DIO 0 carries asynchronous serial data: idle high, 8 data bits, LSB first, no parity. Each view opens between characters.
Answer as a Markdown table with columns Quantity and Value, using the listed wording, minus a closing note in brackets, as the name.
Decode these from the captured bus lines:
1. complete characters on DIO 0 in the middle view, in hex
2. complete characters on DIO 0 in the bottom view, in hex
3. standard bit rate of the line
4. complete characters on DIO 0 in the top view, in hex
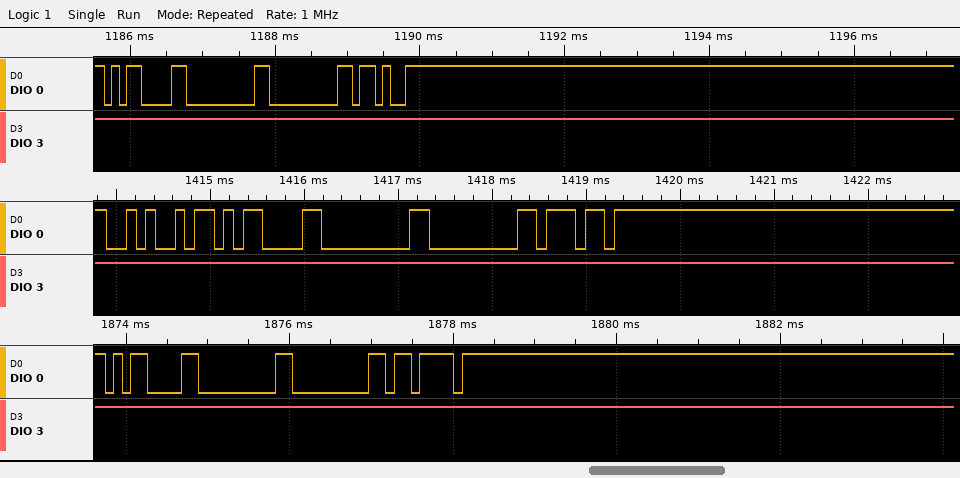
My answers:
| Quantity | Value |
|---|---|
| complete characters on DIO 0 in the middle view, in hex | 4A, 0D, 00, 00, B7 |
| complete characters on DIO 0 in the bottom view, in hex | 0D, 00, 00, 7B |
| standard bit rate of the line | 9600 baud |
| complete characters on DIO 0 in the top view, in hex | 0D, 00, 00, CB |
